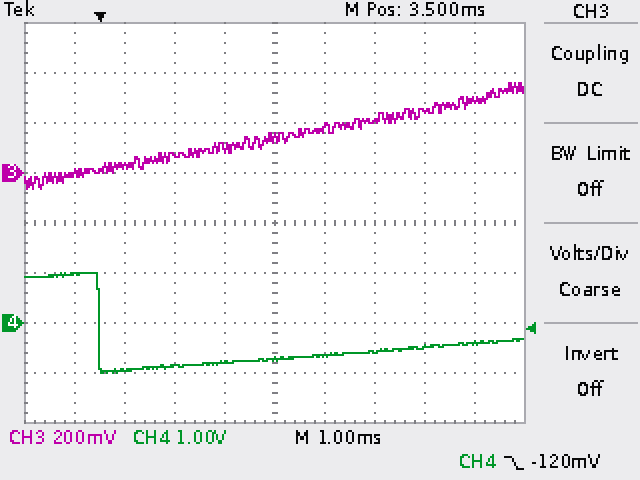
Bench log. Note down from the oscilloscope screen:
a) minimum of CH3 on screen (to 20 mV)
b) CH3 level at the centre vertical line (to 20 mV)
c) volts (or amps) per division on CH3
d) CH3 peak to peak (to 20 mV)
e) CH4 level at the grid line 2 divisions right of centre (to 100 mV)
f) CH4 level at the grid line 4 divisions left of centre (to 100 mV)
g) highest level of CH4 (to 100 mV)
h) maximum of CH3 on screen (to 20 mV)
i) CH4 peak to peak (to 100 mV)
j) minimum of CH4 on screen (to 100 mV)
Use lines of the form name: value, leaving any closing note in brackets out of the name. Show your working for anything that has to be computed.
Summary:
minimum of CH3 on screen: -60 mV
CH3 level at the centre vertical line: 140 mV
volts (or amps) per division on CH3: 200 mV
CH3 peak to peak: 360 mV − (-60 mV) = 420 mV
CH4 level at the grid line 2 divisions right of centre: -600 mV
CH4 level at the grid line 4 divisions left of centre: 1.0 V
highest level of CH4: 1.0 V
maximum of CH3 on screen: 360 mV
CH4 peak to peak: 1.0 V − (-1.0 V) = 2.0 V
minimum of CH4 on screen: -1.0 V
